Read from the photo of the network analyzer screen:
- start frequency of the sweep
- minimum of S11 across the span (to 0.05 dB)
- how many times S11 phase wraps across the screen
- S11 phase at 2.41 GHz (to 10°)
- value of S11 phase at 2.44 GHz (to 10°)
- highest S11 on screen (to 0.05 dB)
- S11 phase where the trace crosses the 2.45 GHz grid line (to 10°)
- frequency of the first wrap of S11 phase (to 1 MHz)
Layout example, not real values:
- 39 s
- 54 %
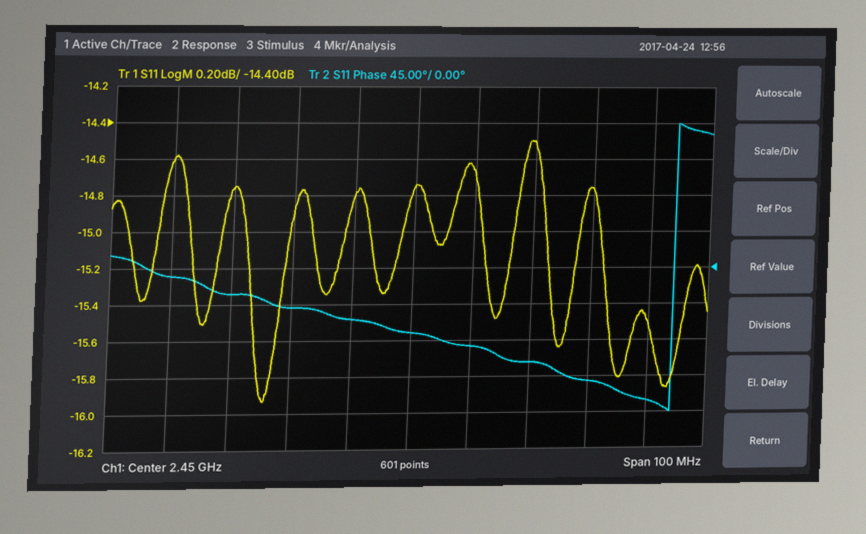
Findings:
- 2.4 GHz
- -15.95 dB
- 1
- -10°
- -60°
- -14.50 dB
- -80°
- 2.494 GHz
